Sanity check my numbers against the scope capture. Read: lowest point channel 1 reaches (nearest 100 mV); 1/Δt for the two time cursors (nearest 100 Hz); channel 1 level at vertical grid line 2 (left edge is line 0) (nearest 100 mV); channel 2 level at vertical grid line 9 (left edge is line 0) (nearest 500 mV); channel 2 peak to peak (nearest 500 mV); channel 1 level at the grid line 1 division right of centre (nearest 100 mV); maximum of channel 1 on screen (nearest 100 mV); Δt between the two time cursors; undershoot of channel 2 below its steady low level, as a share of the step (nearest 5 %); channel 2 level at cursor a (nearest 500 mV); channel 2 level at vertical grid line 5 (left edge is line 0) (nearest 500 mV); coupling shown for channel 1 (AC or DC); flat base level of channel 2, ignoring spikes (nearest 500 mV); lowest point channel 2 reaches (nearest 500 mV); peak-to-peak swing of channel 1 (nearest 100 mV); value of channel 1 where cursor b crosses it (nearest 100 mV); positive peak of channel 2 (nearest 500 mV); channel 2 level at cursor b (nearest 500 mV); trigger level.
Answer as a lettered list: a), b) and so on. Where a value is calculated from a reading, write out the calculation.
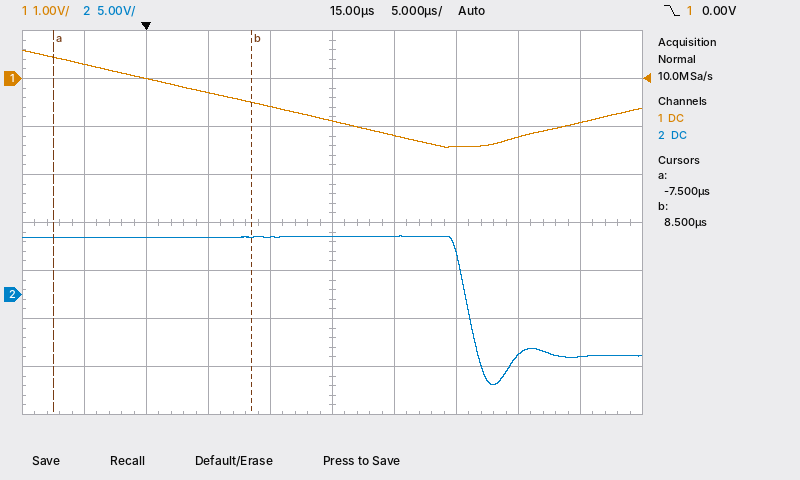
a) -1.4 V
b) 1 / 16.0 µs ≈ 62.5 kHz
c) 0.0 V
d) -6.5 V
e) 6.0 V − (-9.5 V) = 15.5 V
f) -1.2 V
g) 600 mV
h) 8.5 µs − (-7.5 µs) = 16.0 µs
i) 25 %
j) 6.0 V
k) 6.0 V
l) DC
m) -6.5 V
n) -9.5 V
o) 600 mV − (-1.4 V) = 2.0 V
p) -500 mV
q) 6.0 V
r) 6.0 V
s) 0.00 V
